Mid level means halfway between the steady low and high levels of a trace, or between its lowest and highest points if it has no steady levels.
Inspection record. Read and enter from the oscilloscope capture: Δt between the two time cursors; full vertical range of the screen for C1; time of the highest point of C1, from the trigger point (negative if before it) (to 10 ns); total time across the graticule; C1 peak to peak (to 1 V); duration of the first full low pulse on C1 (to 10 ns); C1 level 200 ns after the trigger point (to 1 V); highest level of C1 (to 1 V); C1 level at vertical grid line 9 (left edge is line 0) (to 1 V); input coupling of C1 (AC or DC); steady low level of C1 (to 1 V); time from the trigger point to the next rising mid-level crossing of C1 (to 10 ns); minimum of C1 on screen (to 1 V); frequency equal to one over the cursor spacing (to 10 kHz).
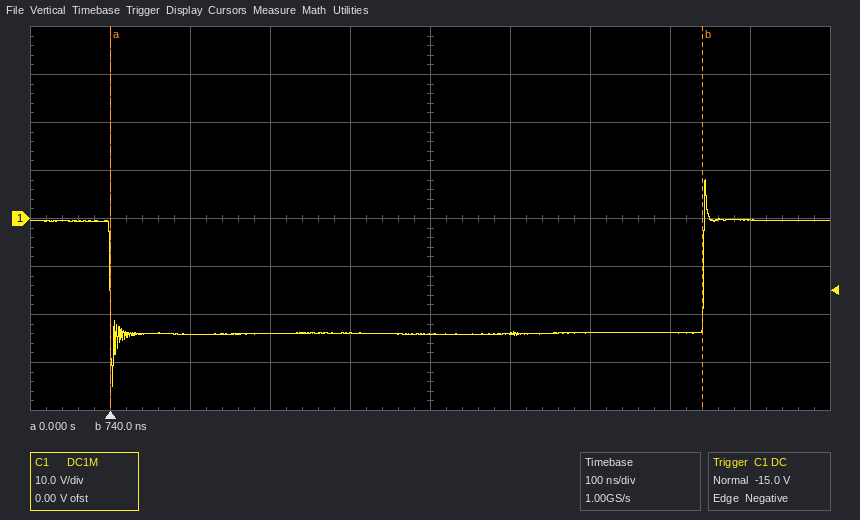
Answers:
740 ns
80 V
+740 ns
1 µs
43 V
740 ns
-24 V
8 V
0 V
DC
-24 V
740 ns
-35 V
1.35 MHz
